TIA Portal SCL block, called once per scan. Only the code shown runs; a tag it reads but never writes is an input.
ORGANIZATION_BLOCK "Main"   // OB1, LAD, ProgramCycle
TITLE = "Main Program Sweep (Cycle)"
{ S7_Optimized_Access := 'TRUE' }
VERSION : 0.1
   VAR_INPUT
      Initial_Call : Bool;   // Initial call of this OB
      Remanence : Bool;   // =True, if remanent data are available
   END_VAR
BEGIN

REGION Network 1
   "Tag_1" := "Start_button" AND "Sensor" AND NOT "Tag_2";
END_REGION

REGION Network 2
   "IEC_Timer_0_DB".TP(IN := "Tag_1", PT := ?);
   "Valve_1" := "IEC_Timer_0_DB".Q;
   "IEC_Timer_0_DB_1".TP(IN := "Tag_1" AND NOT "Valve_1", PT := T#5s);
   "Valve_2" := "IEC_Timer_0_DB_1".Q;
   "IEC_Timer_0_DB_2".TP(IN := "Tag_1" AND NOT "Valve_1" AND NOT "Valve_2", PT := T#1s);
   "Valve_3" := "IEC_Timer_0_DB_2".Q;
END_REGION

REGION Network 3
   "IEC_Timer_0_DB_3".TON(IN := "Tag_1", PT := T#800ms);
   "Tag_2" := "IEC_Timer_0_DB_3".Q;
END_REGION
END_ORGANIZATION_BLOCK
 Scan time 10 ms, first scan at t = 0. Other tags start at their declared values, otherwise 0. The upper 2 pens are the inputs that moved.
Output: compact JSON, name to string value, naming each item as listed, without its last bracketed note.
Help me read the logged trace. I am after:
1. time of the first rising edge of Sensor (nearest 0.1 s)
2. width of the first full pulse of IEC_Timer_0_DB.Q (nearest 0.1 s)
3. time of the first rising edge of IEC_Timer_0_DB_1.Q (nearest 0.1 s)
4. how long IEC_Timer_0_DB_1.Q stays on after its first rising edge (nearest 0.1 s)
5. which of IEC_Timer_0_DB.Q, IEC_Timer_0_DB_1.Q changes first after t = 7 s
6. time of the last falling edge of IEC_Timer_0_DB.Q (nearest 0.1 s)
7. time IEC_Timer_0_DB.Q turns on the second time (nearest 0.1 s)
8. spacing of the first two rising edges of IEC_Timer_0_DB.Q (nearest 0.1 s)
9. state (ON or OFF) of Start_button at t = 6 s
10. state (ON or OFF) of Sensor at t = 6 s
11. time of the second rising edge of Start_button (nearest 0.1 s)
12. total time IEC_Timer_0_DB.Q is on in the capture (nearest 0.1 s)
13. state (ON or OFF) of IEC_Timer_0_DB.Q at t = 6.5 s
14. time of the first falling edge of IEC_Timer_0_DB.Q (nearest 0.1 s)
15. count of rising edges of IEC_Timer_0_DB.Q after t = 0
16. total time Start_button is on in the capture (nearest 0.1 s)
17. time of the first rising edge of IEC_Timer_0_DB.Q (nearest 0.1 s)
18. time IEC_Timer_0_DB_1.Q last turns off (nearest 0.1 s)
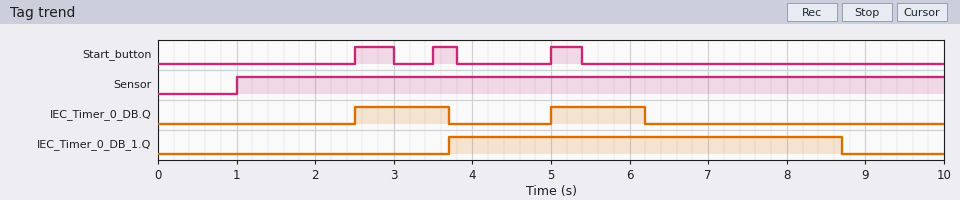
{"time of the first rising edge of Sensor": "1.0 s", "width of the first full pulse of IEC_Timer_0_DB.Q": "1.2 s", "time of the first rising edge of IEC_Timer_0_DB_1.Q": "3.7 s", "how long IEC_Timer_0_DB_1.Q stays on after its first rising edge": "5.0 s", "which of IEC_Timer_0_DB.Q, IEC_Timer_0_DB_1.Q changes first after t = 7 s": "IEC_Timer_0_DB_1.Q", "time of the last falling edge of IEC_Timer_0_DB.Q": "6.2 s", "time IEC_Timer_0_DB.Q turns on the second time": "5.0 s", "spacing of the first two rising edges of IEC_Timer_0_DB.Q": "2.5 s", "state (ON or OFF) of Start_button at t = 6 s": "OFF", "state (ON or OFF) of Sensor at t = 6 s": "ON", "time of the second rising edge of Start_button": "3.5 s", "total time IEC_Timer_0_DB.Q is on in the capture": "2.4 s", "state (ON or OFF) of IEC_Timer_0_DB.Q at t = 6.5 s": "OFF", "time of the first falling edge of IEC_Timer_0_DB.Q": "3.7 s", "count of rising edges of IEC_Timer_0_DB.Q after t = 0": "2", "total time Start_button is on in the capture": "1.2 s", "time of the first rising edge of IEC_Timer_0_DB.Q": "2.5 s", "time IEC_Timer_0_DB_1.Q last turns off": "8.7 s"}
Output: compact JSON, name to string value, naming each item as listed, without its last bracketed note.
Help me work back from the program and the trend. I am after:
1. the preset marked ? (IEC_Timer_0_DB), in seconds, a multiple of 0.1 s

{"the preset marked ? (IEC_Timer_0_DB), in seconds, a multiple of 0.1 s": "1.2 s"}
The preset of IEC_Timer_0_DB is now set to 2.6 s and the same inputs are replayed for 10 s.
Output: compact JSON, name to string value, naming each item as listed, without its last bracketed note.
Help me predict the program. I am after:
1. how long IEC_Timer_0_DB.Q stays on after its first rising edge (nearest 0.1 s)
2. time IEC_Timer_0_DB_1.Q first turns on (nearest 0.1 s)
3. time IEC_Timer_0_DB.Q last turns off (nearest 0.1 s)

{"how long IEC_Timer_0_DB.Q stays on after its first rising edge": "2.6 s", "time IEC_Timer_0_DB_1.Q first turns on": "5.1 s", "time IEC_Timer_0_DB.Q last turns off": "5.1 s"}
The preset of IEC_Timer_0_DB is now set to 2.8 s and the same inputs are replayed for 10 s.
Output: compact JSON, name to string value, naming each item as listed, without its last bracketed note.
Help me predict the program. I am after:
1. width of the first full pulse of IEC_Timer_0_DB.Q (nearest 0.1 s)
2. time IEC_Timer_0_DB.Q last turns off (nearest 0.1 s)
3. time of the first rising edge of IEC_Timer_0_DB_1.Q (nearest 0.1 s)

{"width of the first full pulse of IEC_Timer_0_DB.Q": "2.8 s", "time IEC_Timer_0_DB.Q last turns off": "5.3 s", "time of the first rising edge of IEC_Timer_0_DB_1.Q": "5.3 s"}
